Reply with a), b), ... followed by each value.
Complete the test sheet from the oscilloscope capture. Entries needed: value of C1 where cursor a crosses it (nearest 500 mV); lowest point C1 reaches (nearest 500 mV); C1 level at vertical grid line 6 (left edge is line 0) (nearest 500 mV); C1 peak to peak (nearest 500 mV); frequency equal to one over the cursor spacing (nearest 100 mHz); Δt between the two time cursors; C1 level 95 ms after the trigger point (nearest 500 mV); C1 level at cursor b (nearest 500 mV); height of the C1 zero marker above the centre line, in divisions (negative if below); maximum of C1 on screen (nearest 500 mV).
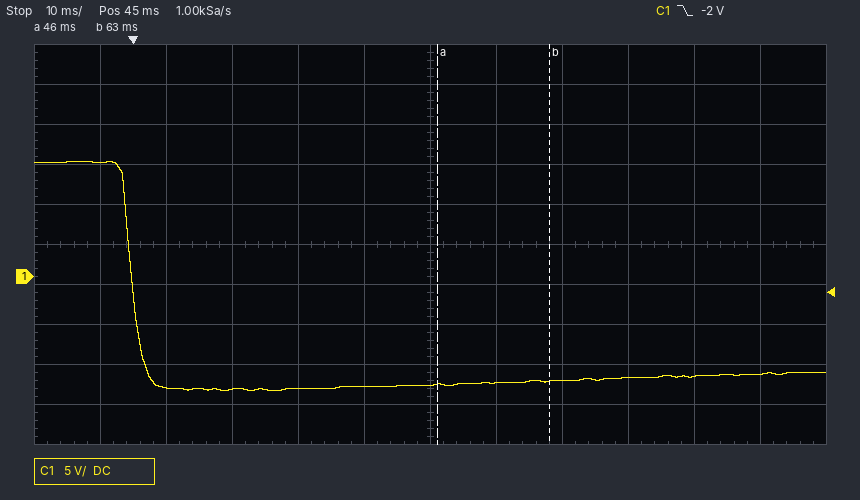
a) -13.5 V
b) -14.0 V
c) -13.5 V
d) 28.5 V
e) 58.8 Hz
f) 17 ms
g) -12.0 V
h) -13.0 V
i) -0.8 div
j) 14.5 V
